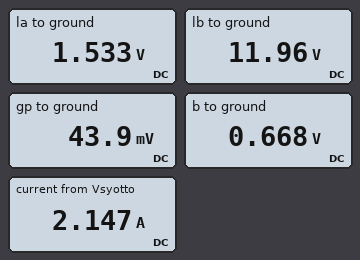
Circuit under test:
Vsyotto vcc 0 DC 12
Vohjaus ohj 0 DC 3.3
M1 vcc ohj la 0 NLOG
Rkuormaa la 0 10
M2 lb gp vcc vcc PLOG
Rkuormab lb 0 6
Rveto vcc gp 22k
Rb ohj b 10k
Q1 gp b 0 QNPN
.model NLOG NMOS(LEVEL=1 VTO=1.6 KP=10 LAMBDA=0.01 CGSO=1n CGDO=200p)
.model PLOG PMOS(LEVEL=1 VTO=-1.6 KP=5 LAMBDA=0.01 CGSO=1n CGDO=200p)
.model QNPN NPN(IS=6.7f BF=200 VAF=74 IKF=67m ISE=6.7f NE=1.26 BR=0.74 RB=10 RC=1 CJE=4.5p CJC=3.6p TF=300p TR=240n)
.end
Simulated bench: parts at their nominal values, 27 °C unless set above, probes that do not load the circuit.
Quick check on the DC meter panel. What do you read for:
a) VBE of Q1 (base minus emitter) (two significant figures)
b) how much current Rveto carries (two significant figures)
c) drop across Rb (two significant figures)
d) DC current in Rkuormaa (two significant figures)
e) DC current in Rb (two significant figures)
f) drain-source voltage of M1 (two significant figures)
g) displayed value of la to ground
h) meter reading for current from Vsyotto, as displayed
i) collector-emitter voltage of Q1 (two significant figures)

670 mV
540 µA
2.6 V
150 mA
260 µA
10 V
1.533 V
2.147 A
44 mV
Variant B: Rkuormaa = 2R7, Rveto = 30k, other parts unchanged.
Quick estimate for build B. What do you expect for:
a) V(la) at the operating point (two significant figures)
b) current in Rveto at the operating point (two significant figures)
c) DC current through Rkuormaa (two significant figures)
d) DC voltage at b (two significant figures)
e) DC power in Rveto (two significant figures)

1.4 V
400 µA
520 mA
660 mV
4.8 mW
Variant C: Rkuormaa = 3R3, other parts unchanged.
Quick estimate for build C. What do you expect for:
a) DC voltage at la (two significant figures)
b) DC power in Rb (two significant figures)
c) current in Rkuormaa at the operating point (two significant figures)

1.4 V
690 µW
430 mA
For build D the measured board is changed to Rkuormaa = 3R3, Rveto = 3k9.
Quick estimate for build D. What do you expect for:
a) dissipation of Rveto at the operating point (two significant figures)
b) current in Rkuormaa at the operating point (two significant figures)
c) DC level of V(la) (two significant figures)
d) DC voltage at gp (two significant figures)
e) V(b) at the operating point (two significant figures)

36 mW
430 mA
1.4 V
83 mV
700 mV
